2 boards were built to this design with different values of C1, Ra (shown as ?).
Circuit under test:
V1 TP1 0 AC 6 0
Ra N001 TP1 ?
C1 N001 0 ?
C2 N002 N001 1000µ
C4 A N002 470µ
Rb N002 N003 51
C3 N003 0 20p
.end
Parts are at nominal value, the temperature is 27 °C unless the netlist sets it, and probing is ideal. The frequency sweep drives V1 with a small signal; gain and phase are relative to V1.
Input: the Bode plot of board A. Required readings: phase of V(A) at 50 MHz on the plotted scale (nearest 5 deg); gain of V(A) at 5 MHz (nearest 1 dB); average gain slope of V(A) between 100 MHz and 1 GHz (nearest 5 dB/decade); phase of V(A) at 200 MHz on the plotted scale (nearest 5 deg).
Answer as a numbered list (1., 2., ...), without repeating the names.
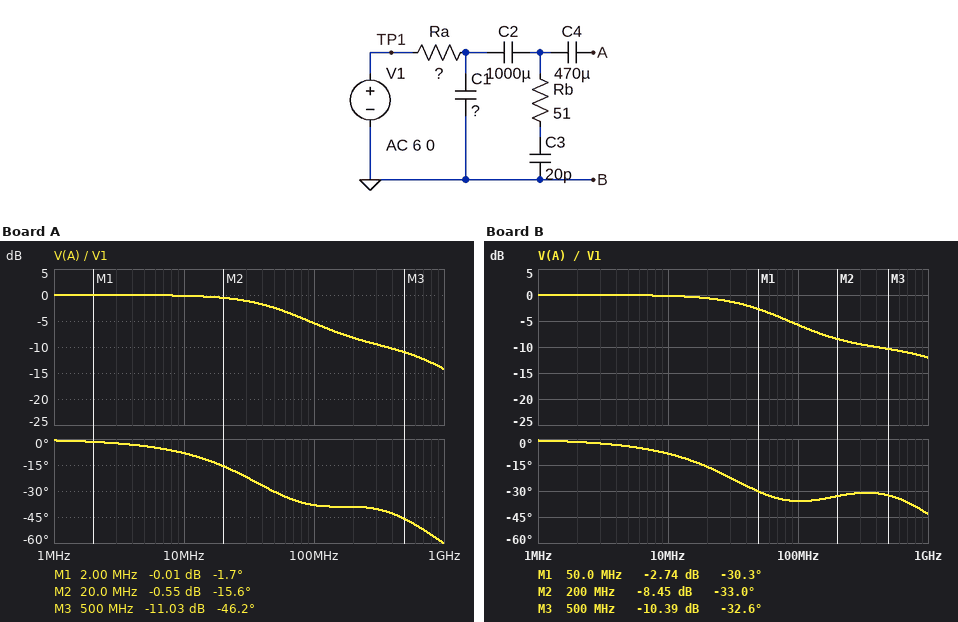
1. -30 deg
2. 0 dB
3. -10 dB/decade
4. -40 deg
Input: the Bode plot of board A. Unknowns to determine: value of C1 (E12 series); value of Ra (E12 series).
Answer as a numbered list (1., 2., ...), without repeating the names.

1. 8.2 pF
2. 82 Ω
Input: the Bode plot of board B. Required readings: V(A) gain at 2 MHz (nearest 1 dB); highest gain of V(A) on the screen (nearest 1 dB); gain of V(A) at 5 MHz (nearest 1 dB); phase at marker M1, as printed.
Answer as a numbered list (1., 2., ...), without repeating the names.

1. 0 dB
2. 0 dB
3. 0 dB
4. -30.3 deg
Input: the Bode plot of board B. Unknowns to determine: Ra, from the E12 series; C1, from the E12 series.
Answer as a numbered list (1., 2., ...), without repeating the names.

1. 100 Ω
2. 3.9 pF
